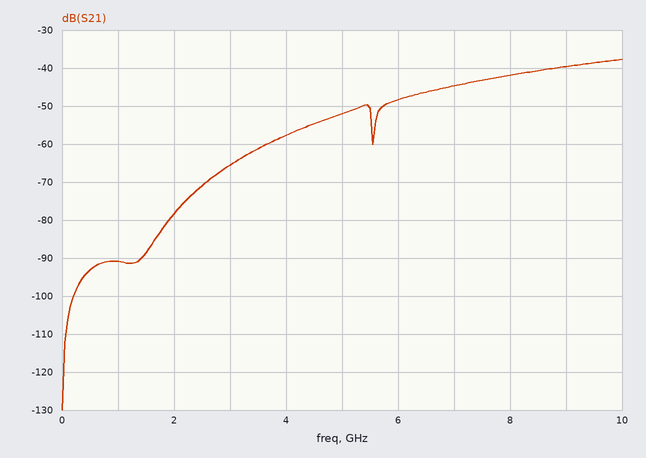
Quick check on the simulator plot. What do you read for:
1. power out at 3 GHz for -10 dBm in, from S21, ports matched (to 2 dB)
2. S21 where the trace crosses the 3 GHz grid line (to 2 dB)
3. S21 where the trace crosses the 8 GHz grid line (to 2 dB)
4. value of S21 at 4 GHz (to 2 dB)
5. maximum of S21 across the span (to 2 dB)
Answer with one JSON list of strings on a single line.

["-76 dBm", "-66 dB", "-42 dB", "-58 dB", "-38 dB"]
